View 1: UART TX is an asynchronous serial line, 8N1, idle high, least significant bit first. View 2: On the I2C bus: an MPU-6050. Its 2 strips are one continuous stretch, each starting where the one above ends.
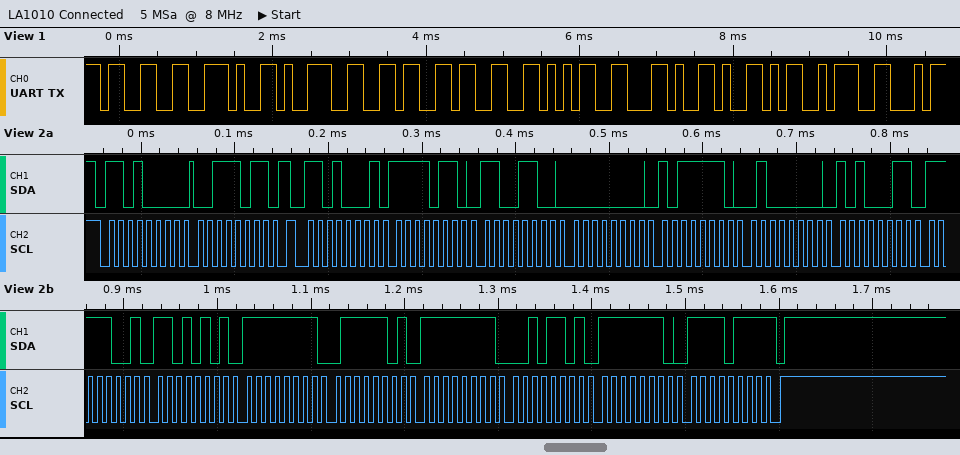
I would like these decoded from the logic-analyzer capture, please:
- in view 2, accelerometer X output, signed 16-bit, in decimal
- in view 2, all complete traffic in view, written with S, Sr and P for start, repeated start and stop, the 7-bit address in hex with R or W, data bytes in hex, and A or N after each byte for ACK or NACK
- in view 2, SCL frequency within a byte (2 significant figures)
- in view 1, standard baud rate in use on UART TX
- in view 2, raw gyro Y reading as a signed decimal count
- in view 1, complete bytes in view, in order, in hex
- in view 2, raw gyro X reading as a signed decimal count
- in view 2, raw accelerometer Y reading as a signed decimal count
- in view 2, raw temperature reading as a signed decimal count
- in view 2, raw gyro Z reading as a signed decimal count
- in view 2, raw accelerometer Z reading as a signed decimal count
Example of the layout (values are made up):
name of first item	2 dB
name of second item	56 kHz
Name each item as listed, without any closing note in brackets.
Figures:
in view 2, accelerometer X output, signed 16-bit, in decimal	-2356
in view 2, all complete traffic in view, written with S, Sr and P for start, repeated start and stop, the 7-bit address in hex with R or W, data bytes in hex, and A or N after each byte for ACK or NACK	S 68W A 3B A Sr 68R A F6 A CC A 00 A BE A 40 A A3 A F9 A D5 A FF A 7D A FF A 2D A FE A F7 N P
in view 2, SCL frequency within a byte	100 kHz
in view 1, standard baud rate in use on UART TX	9600 baud
in view 2, raw gyro Y reading as a signed decimal count	-211
in view 1, complete bytes in view, in order, in hex	0x33 0x2E 0x39 0x36 0x33 0x35 0x2C 0x59 0x3A
in view 2, raw gyro X reading as a signed decimal count	-131
in view 2, raw accelerometer Y reading as a signed decimal count	190
in view 2, raw temperature reading as a signed decimal count	-1579
in view 2, raw gyro Z reading as a signed decimal count	-265
in view 2, raw accelerometer Z reading as a signed decimal count	16547
